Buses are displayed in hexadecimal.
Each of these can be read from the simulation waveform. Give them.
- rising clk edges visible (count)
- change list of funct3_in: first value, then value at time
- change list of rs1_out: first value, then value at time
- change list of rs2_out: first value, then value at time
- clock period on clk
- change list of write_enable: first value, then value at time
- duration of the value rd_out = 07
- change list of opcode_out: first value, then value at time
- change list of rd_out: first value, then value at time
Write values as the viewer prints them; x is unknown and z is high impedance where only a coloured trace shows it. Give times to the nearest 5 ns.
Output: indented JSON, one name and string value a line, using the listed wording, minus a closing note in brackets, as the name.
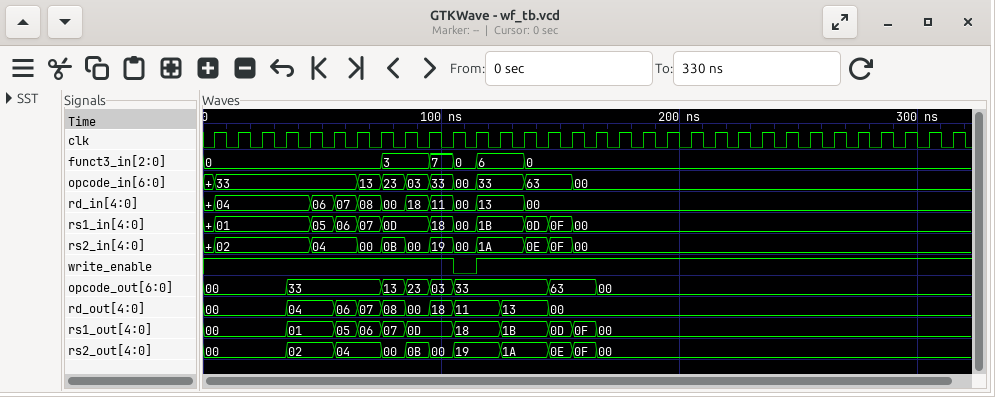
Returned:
{
  "rising clk edges visible": "32",
  "change list of funct3_in: first value, then value at time": "0, 3 at 75 ns, 7 at 95 ns, 0 at 105 ns, 6 at 115 ns, 0 at 135 ns",
  "change list of rs1_out: first value, then value at time": "00, 01 at 35 ns, 05 at 55 ns, 06 at 65 ns, 07 at 75 ns, 0D at 85 ns, 18 at 105 ns, 1B at 125 ns, 0D at 145 ns, 0F at 155 ns, 00 at 165 ns",
  "change list of rs2_out: first value, then value at time": "00, 02 at 35 ns, 04 at 55 ns, 00 at 75 ns, 0B at 85 ns, 00 at 95 ns, 19 at 105 ns, 1A at 125 ns, 0E at 145 ns, 0F at 155 ns, 00 at 165 ns",
  "clock period on clk": "10 ns",
  "change list of write_enable: first value, then value at time": "1, 0 at 105 ns, 1 at 115 ns",
  "duration of the value rd_out = 07": "10 ns",
  "change list of opcode_out: first value, then value at time": "00, 33 at 35 ns, 13 at 75 ns, 23 at 85 ns, 03 at 95 ns, 33 at 105 ns, 63 at 145 ns, 00 at 165 ns",
  "change list of rd_out: first value, then value at time": "00, 04 at 35 ns, 06 at 55 ns, 07 at 65 ns, 08 at 75 ns, 00 at 85 ns, 18 at 95 ns, 11 at 105 ns, 13 at 125 ns, 00 at 145 ns"
}
